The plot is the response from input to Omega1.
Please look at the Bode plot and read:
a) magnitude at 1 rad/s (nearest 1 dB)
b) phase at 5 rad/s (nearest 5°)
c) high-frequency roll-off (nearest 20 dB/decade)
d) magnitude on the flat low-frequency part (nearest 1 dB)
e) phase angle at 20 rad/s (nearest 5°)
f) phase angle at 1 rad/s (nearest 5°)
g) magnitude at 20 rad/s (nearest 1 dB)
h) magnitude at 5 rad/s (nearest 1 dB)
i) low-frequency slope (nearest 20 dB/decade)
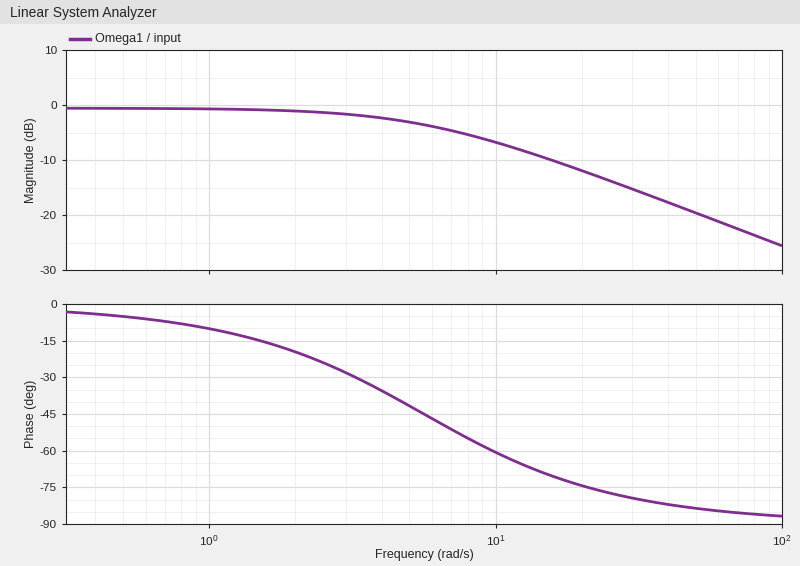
-1 dB
-40°
-20 dB/decade
-1 dB
-75°
-10°
-12 dB
-3 dB
0 dB/decade
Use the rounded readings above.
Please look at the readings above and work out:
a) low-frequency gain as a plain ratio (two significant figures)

0.89
